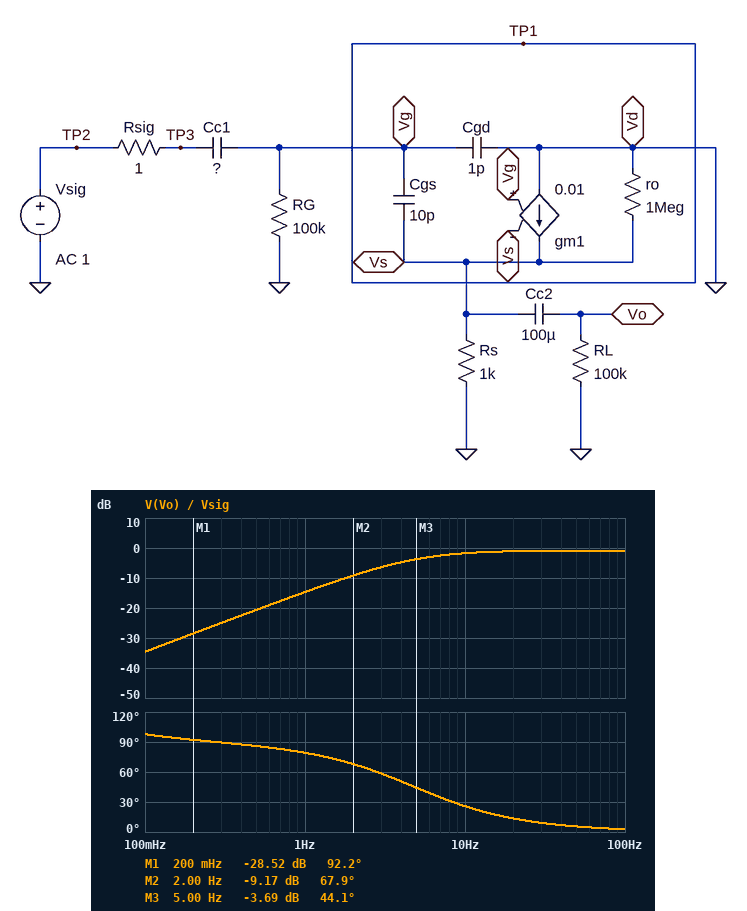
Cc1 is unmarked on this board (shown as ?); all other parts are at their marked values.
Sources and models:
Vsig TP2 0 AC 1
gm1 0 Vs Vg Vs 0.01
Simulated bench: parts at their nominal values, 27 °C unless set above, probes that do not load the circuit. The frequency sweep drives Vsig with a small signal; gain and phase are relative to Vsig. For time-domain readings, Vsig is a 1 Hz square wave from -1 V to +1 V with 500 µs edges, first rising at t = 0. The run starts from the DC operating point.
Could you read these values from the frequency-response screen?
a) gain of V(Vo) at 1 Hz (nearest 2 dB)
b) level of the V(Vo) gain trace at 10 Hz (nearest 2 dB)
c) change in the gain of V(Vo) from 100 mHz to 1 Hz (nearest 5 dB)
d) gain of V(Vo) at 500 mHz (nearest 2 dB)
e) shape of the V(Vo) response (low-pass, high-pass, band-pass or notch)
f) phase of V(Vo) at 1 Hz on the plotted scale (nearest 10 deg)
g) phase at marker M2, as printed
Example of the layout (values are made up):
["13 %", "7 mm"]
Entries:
["-14 dB", "-2 dB", "20 dB", "-20 dB", "high-pass", "80 deg", "67.9 deg"]
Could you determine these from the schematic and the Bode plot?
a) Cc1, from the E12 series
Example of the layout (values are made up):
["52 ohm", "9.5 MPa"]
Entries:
["330 nF"]
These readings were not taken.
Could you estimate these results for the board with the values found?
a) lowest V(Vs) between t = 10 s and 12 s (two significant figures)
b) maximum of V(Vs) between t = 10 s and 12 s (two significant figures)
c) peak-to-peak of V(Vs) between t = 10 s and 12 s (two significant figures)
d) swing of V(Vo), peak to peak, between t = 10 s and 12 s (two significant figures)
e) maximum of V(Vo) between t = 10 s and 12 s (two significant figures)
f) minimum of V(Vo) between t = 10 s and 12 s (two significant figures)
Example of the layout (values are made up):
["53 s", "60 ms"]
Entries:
["-1.8 V", "1.8 V", "3.6 V", "3.6 V", "1.8 V", "-1.8 V"]
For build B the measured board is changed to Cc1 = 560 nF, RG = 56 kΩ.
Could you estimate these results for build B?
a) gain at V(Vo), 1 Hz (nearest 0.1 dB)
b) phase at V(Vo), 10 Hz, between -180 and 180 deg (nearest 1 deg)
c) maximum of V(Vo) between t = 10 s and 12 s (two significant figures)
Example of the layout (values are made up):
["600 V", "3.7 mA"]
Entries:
["-15.1 dB", "27 deg", "1.8 V"]
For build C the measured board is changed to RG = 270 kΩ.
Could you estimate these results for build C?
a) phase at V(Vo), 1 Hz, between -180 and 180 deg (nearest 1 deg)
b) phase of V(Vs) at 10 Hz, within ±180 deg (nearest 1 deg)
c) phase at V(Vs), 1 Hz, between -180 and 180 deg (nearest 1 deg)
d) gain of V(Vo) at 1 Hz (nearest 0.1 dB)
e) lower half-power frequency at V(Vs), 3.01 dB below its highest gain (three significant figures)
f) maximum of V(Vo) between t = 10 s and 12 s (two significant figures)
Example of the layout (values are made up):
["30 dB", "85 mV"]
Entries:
["62 deg", "10 deg", "61 deg", "-7.1 dB", "1.79 Hz", "1.8 V"]
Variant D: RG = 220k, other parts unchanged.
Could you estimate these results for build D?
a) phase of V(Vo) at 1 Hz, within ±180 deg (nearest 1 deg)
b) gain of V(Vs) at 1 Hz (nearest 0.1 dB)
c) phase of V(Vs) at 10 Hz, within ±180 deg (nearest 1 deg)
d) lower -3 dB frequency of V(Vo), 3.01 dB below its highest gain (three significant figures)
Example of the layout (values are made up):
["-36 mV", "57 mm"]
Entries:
["66 deg", "-8.5 dB", "12 deg", "2.19 Hz"]
